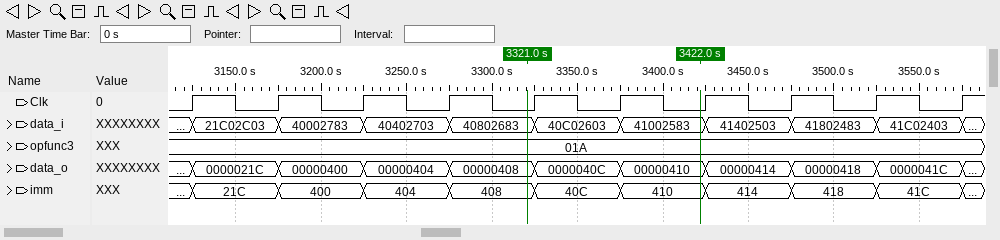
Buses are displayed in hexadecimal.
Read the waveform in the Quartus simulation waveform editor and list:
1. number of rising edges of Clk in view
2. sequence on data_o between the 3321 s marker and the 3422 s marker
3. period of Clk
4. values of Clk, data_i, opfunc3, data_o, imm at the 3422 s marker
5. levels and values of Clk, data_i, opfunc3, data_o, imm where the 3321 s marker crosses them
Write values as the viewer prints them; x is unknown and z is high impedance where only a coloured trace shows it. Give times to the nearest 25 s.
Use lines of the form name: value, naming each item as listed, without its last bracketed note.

number of rising edges of Clk in view: 10
sequence on data_o between the 3321 s marker and the 3422 s marker: 00000408, 0000040C, 00000410
period of Clk: 50 s
values of Clk, data_i, opfunc3, data_o, imm at the 3422 s marker: Clk=0, data_i=41002583, opfunc3=01A, data_o=00000410, imm=410
levels and values of Clk, data_i, opfunc3, data_o, imm where the 3321 s marker crosses them: Clk=0, data_i=40802683, opfunc3=01A, data_o=00000408, imm=408
